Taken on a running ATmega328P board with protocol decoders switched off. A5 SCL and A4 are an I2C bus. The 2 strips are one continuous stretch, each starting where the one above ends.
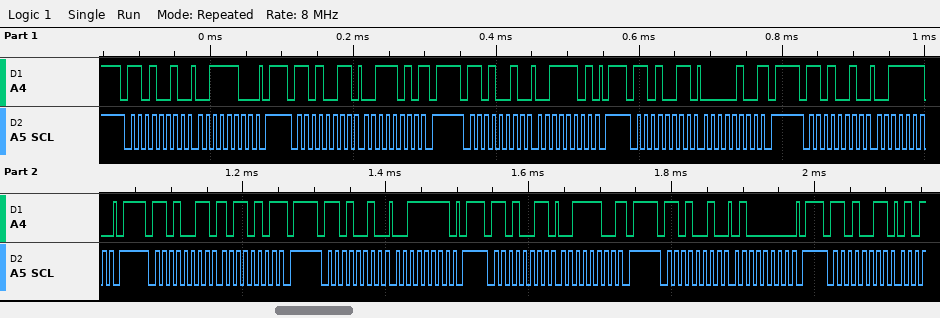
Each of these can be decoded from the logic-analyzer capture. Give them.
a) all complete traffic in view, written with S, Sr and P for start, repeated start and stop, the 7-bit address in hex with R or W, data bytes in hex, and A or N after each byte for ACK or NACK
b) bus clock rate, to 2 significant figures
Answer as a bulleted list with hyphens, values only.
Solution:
- S 69W A 3C A P S 69R A 3A N P S 69W A 3D A P S 69R A 04 N P S 69W A 3E A P S 69R A B5 N P S 69W A 3F A P S 69R A 3C N P S 69W A 40 A P S 69R A
- 100 kHz
